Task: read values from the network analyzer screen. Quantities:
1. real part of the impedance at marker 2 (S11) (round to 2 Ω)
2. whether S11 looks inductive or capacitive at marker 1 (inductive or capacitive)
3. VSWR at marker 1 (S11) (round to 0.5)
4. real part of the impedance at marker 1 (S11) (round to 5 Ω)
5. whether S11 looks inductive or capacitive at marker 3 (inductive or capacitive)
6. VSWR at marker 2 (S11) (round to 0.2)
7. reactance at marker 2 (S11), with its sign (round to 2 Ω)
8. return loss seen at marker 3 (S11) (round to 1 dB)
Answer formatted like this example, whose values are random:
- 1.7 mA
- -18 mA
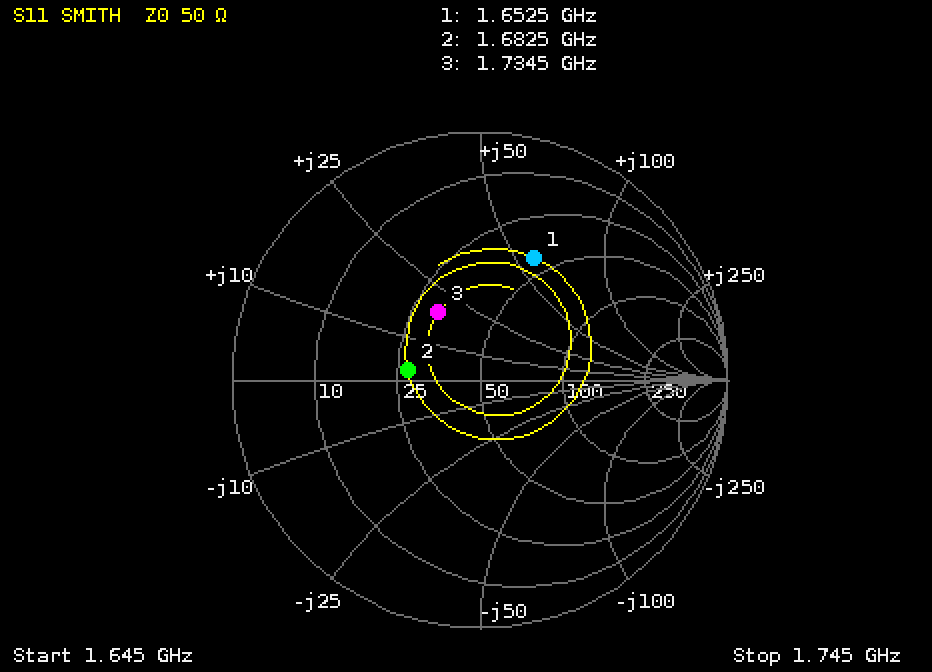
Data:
- 28 Ω
- inductive
- 3.5
- 40 Ω
- inductive
- 1.8
- +2 Ω
- 10 dB
